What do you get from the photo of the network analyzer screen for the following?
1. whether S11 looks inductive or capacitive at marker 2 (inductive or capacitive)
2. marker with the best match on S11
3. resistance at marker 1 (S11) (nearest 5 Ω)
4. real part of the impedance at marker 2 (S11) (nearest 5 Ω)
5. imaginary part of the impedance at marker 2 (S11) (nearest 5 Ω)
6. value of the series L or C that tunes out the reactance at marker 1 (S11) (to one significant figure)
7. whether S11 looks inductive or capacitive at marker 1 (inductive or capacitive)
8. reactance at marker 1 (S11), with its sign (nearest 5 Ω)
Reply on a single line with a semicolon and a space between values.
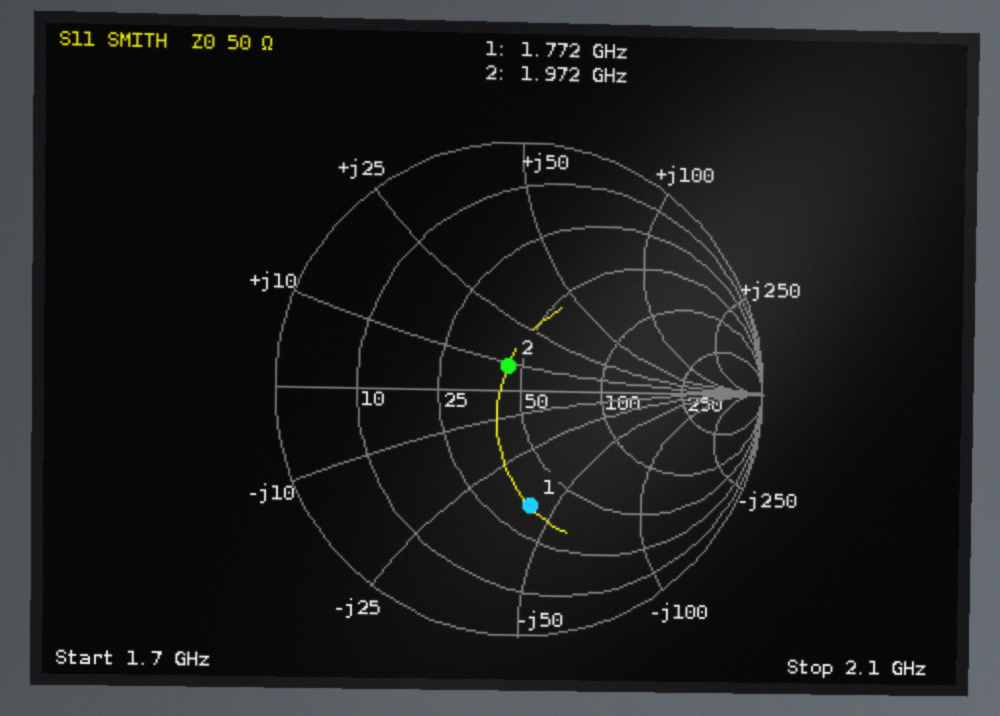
inductive; marker 2; 35 Ω; 45 Ω; +10 Ω; 4 nH; capacitive; -40 Ω
